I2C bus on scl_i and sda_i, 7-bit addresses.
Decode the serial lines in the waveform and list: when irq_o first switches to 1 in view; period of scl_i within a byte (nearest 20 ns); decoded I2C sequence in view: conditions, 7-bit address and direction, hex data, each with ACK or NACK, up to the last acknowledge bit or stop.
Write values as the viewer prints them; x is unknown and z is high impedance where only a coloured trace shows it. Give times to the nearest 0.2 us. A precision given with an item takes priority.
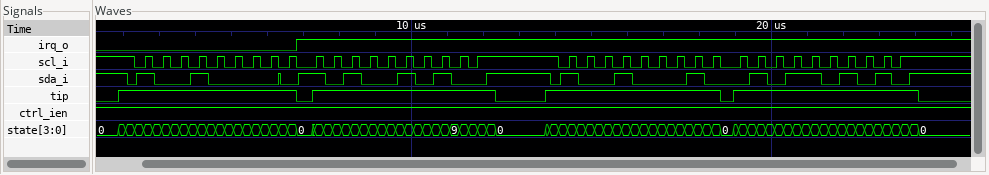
6.8 us
500 ns
start, address 48 write ACK, A5 ACK, stop, start, address 48 read ACK, 5A NACK, stop
